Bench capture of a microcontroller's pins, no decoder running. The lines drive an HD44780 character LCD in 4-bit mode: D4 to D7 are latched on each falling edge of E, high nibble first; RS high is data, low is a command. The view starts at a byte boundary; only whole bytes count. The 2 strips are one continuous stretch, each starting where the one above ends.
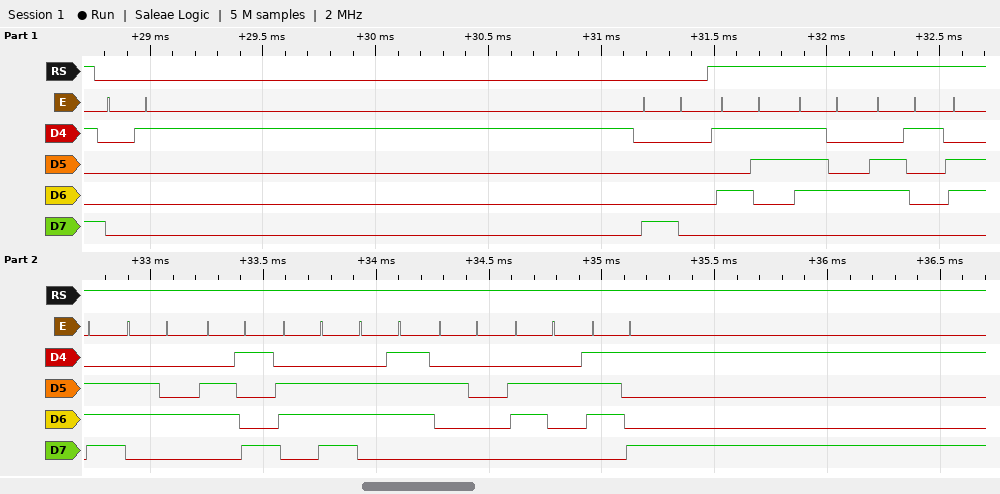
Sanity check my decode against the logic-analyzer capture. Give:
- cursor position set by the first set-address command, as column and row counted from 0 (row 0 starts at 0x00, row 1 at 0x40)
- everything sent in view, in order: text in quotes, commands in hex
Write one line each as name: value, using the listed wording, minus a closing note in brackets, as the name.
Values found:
cursor position set by the first set-address command, as column and row counted from 0: column 0, row 0
everything sent in view, in order: text in quotes, commands in hex: 0x01 0x80 "Standing by"
